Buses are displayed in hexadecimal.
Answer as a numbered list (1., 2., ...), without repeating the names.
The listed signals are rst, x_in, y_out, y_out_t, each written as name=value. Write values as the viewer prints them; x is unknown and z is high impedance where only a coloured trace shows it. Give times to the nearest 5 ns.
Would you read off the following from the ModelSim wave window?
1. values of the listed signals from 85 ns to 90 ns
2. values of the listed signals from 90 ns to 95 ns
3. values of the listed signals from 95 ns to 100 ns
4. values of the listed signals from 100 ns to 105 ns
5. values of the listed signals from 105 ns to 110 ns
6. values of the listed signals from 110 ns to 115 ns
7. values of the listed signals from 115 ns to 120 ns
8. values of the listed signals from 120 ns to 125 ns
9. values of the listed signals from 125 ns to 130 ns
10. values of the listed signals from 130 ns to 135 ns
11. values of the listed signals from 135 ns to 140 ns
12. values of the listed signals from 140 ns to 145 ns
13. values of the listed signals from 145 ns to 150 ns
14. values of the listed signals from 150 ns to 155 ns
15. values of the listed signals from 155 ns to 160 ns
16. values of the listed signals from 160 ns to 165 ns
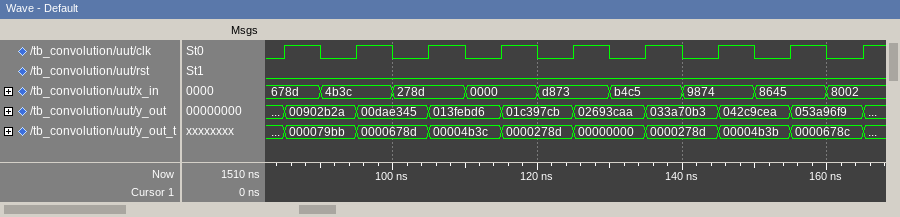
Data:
1. rst=0, x_in=678d, y_out=00902b2a, y_out_t=000079bb
2. rst=0, x_in=4b3c, y_out=00902b2a, y_out_t=000079bb
3. rst=0, x_in=4b3c, y_out=00dae345, y_out_t=0000678d
4. rst=0, x_in=278d, y_out=00dae345, y_out_t=0000678d
5. rst=0, x_in=278d, y_out=013febd6, y_out_t=00004b3c
6. rst=0, x_in=0000, y_out=013febd6, y_out_t=00004b3c
7. rst=0, x_in=0000, y_out=01c397cb, y_out_t=0000278d
8. rst=0, x_in=d873, y_out=01c397cb, y_out_t=0000278d
9. rst=0, x_in=d873, y_out=02693caa, y_out_t=00000000
10. rst=0, x_in=b4c5, y_out=02693caa, y_out_t=00000000
11. rst=0, x_in=b4c5, y_out=033a70b3, y_out_t=0000278d
12. rst=0, x_in=9874, y_out=033a70b3, y_out_t=0000278d
13. rst=0, x_in=9874, y_out=042c9cea, y_out_t=00004b3b
14. rst=0, x_in=8645, y_out=042c9cea, y_out_t=00004b3b
15. rst=0, x_in=8645, y_out=053a96f9, y_out_t=0000678c
16. rst=0, x_in=8002, y_out=053a96f9, y_out_t=0000678c
